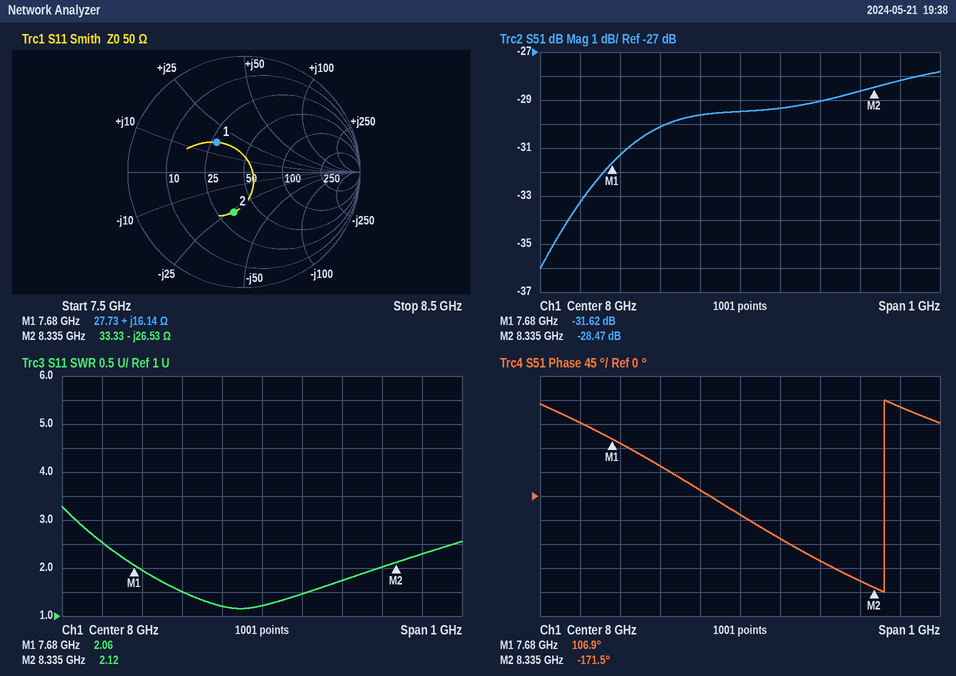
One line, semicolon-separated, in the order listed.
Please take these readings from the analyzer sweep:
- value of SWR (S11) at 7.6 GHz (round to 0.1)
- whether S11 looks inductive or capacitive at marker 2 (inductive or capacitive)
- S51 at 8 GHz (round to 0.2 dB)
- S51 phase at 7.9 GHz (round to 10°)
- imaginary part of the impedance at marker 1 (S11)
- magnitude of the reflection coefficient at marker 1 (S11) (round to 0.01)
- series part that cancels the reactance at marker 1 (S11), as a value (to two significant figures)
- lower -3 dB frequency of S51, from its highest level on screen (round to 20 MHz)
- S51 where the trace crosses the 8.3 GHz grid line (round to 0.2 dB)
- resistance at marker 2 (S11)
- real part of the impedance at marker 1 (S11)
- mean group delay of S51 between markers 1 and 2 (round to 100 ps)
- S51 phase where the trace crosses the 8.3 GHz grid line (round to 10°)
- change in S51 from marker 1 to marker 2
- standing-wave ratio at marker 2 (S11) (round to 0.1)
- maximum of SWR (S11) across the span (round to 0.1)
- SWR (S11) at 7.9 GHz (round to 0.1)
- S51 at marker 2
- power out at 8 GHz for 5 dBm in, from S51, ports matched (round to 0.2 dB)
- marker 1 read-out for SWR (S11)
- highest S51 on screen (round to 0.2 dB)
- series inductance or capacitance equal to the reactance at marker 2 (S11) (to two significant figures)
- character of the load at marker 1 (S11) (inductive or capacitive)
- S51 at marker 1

2.5; capacitive; -29.4 dB; 10°; +16.14 Ω; 0.35; 1.3 pF; 7.74 GHz; -28.6 dB; 33.33 Ω; 27.73 Ω; 1.2 ns; -160°; 3.15 dB; 2.1; 3.3; 1.2; -28.47 dB; -24.4 dBm; 2.06; -27.8 dB; 720 fF; inductive; -31.62 dB
